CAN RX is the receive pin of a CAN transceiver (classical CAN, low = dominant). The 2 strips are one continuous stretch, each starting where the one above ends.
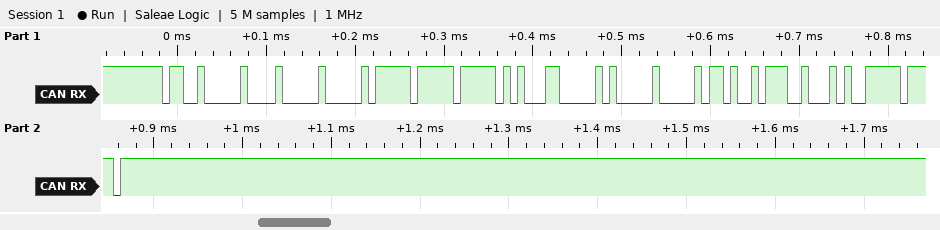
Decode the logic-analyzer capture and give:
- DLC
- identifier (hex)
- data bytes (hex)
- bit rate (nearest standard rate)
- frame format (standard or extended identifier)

8
0x640
00 FF FF 46 04 00 69 72
125 kbit/s
standard
